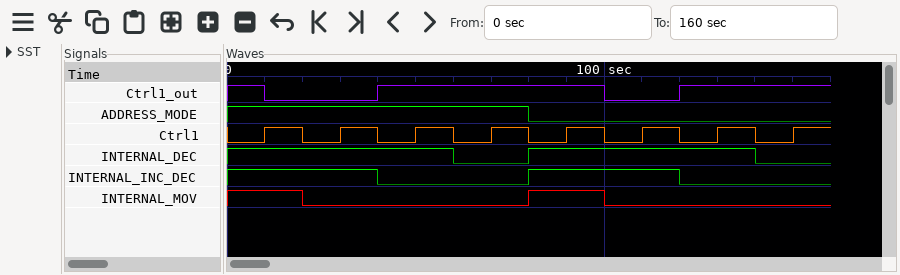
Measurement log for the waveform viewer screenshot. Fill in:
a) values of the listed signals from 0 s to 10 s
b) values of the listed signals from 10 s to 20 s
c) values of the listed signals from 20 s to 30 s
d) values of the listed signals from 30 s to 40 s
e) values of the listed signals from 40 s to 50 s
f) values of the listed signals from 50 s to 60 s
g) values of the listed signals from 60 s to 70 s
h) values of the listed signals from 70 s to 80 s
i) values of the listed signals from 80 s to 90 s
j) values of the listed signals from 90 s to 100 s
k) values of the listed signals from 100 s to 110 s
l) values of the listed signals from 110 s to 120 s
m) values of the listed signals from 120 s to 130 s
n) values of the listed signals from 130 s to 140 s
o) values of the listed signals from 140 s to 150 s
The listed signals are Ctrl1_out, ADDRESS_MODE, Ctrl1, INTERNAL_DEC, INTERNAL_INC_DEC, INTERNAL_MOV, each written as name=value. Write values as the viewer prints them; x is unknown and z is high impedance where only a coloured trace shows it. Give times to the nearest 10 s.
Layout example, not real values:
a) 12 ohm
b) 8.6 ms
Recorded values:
a) Ctrl1_out=1, ADDRESS_MODE=1, Ctrl1=0, INTERNAL_DEC=1, INTERNAL_INC_DEC=1, INTERNAL_MOV=1
b) Ctrl1_out=0, ADDRESS_MODE=1, Ctrl1=1, INTERNAL_DEC=1, INTERNAL_INC_DEC=1, INTERNAL_MOV=1
c) Ctrl1_out=0, ADDRESS_MODE=1, Ctrl1=0, INTERNAL_DEC=1, INTERNAL_INC_DEC=1, INTERNAL_MOV=0
d) Ctrl1_out=0, ADDRESS_MODE=1, Ctrl1=1, INTERNAL_DEC=1, INTERNAL_INC_DEC=1, INTERNAL_MOV=0
e) Ctrl1_out=1, ADDRESS_MODE=1, Ctrl1=0, INTERNAL_DEC=1, INTERNAL_INC_DEC=0, INTERNAL_MOV=0
f) Ctrl1_out=1, ADDRESS_MODE=1, Ctrl1=1, INTERNAL_DEC=1, INTERNAL_INC_DEC=0, INTERNAL_MOV=0
g) Ctrl1_out=1, ADDRESS_MODE=1, Ctrl1=0, INTERNAL_DEC=0, INTERNAL_INC_DEC=0, INTERNAL_MOV=0
h) Ctrl1_out=1, ADDRESS_MODE=1, Ctrl1=1, INTERNAL_DEC=0, INTERNAL_INC_DEC=0, INTERNAL_MOV=0
i) Ctrl1_out=1, ADDRESS_MODE=0, Ctrl1=0, INTERNAL_DEC=1, INTERNAL_INC_DEC=1, INTERNAL_MOV=1
j) Ctrl1_out=1, ADDRESS_MODE=0, Ctrl1=1, INTERNAL_DEC=1, INTERNAL_INC_DEC=1, INTERNAL_MOV=1
k) Ctrl1_out=0, ADDRESS_MODE=0, Ctrl1=0, INTERNAL_DEC=1, INTERNAL_INC_DEC=1, INTERNAL_MOV=0
l) Ctrl1_out=0, ADDRESS_MODE=0, Ctrl1=1, INTERNAL_DEC=1, INTERNAL_INC_DEC=1, INTERNAL_MOV=0
m) Ctrl1_out=1, ADDRESS_MODE=0, Ctrl1=0, INTERNAL_DEC=1, INTERNAL_INC_DEC=0, INTERNAL_MOV=0
n) Ctrl1_out=1, ADDRESS_MODE=0, Ctrl1=1, INTERNAL_DEC=1, INTERNAL_INC_DEC=0, INTERNAL_MOV=0
o) Ctrl1_out=1, ADDRESS_MODE=0, Ctrl1=0, INTERNAL_DEC=0, INTERNAL_INC_DEC=0, INTERNAL_MOV=0
